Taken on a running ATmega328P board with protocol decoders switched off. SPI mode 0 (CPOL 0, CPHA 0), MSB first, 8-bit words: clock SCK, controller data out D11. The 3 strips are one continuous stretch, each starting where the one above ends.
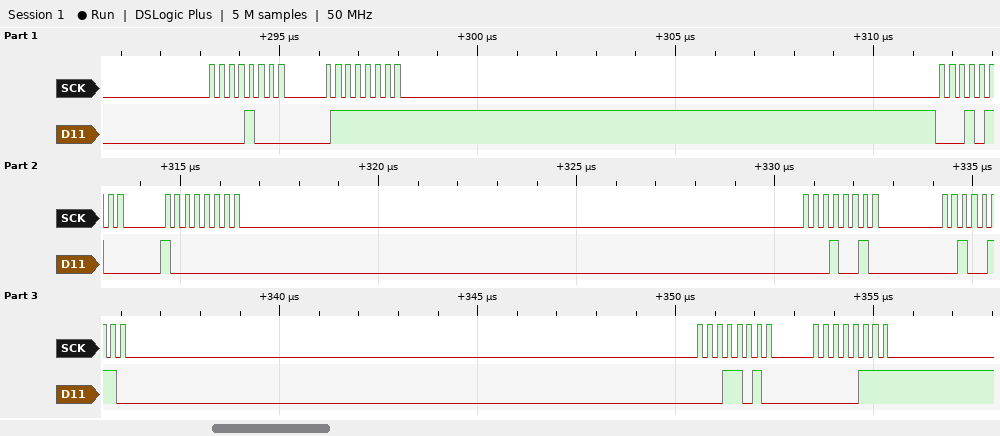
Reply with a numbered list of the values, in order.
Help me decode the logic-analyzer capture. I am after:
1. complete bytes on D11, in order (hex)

1. 08 7F 14 80 12 26 1A 07
